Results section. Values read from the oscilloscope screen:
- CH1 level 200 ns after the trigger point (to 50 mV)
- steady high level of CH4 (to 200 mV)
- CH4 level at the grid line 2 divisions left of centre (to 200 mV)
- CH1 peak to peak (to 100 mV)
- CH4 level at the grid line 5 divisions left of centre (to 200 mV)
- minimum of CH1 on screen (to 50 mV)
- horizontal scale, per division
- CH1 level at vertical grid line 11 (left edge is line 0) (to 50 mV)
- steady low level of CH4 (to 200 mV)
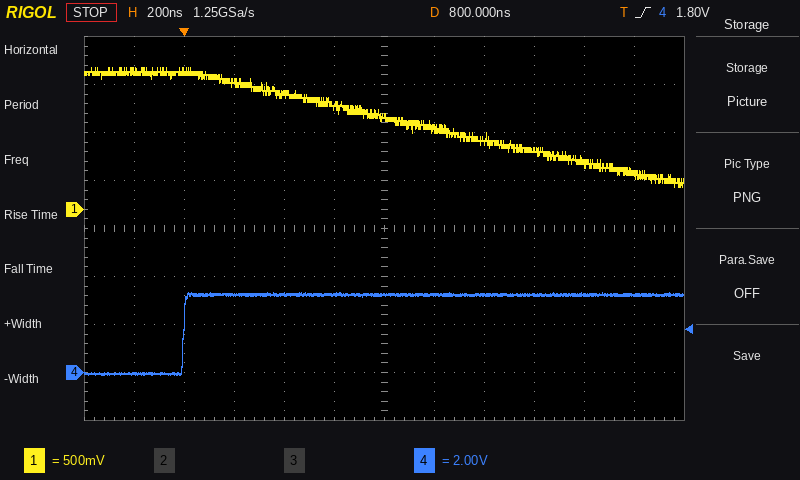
1.30 V
3.2 V
3.2 V
1.20 V
0.0 V
250 mV
200 ns
350 mV
0.0 V
